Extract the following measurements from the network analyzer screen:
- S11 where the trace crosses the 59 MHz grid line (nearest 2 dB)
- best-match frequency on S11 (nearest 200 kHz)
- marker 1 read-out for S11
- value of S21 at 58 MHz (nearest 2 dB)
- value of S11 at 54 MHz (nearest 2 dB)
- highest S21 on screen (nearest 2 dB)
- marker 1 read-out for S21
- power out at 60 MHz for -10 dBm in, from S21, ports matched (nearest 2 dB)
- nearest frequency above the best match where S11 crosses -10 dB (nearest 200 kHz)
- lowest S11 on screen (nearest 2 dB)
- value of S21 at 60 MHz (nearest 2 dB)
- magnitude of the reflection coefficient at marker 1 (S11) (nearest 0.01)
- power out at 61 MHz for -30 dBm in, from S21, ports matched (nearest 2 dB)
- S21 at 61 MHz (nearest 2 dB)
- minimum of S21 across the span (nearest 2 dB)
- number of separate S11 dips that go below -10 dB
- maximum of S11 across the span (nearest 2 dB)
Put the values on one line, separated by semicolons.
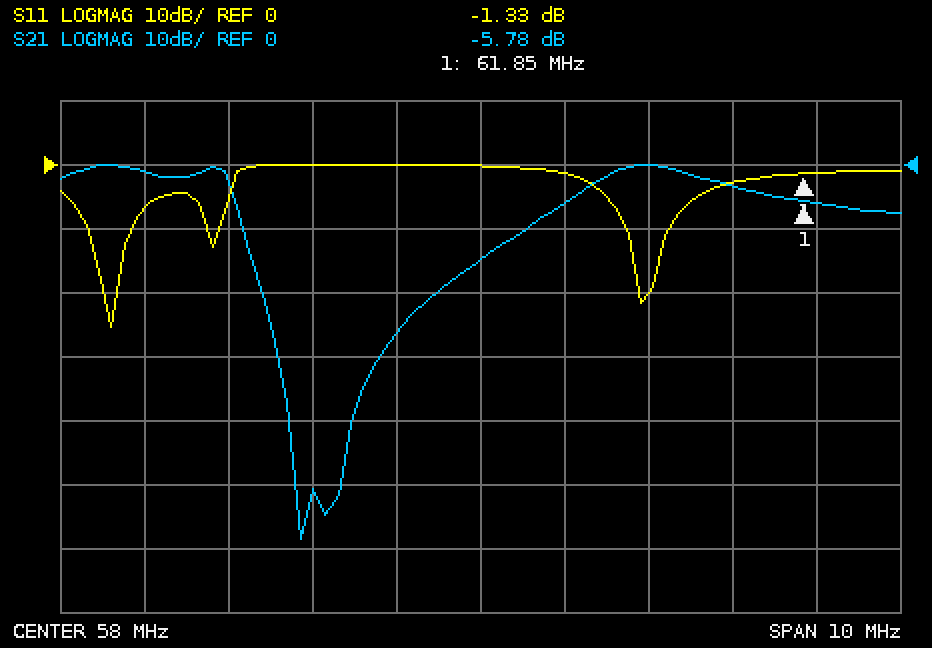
-2 dB; 53.6 MHz; -1.33 dB; -14 dB; -6 dB; 0 dB; -5.78 dB; -10 dBm; 53.8 MHz; -26 dB; 0 dB; 0.86; -34 dBm; -4 dB; -58 dB; 3; 0 dB
